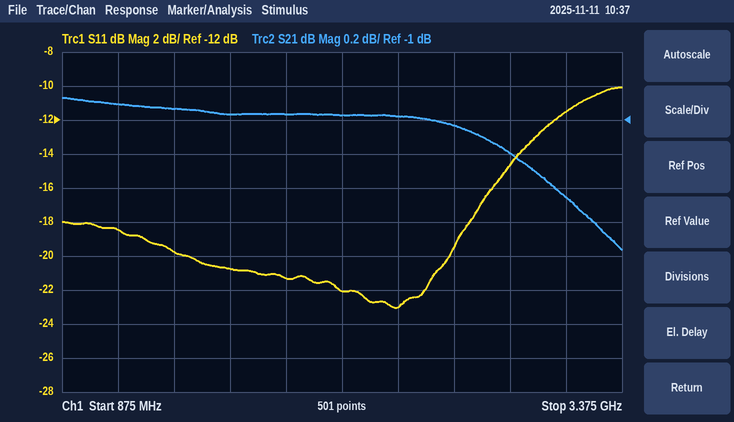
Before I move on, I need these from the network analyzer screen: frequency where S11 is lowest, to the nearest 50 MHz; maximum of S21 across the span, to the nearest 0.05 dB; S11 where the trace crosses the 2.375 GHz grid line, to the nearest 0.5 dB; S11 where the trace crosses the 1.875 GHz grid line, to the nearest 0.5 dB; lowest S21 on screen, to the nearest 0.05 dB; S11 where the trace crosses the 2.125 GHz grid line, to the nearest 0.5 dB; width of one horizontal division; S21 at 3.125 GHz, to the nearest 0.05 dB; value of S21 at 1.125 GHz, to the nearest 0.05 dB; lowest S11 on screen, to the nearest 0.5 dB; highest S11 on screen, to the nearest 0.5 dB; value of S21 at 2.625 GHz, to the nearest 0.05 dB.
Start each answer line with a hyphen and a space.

- 2.35 GHz
- -0.85 dB
- -23.0 dB
- -21.5 dB
- -1.75 dB
- -22.0 dB
- 250 MHz
- -1.45 dB
- -0.90 dB
- -23.0 dB
- -10.0 dB
- -1.05 dB
